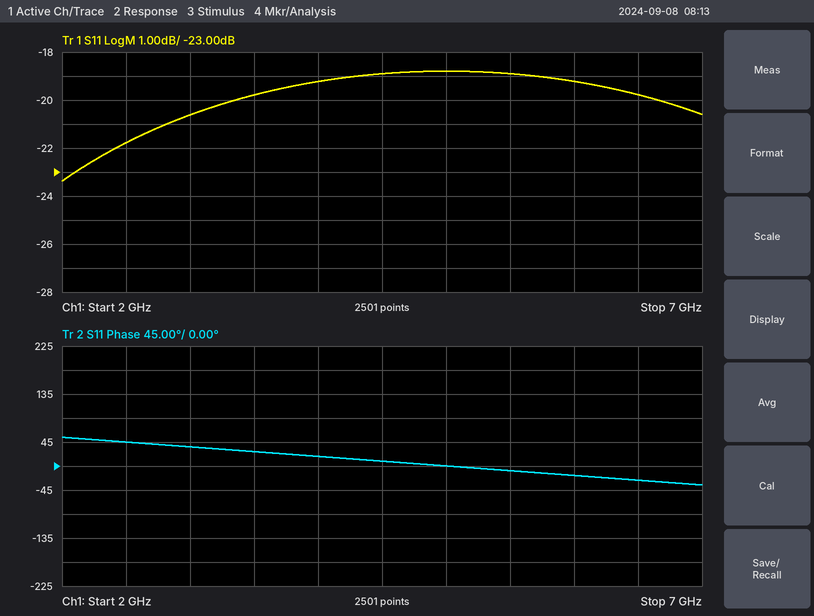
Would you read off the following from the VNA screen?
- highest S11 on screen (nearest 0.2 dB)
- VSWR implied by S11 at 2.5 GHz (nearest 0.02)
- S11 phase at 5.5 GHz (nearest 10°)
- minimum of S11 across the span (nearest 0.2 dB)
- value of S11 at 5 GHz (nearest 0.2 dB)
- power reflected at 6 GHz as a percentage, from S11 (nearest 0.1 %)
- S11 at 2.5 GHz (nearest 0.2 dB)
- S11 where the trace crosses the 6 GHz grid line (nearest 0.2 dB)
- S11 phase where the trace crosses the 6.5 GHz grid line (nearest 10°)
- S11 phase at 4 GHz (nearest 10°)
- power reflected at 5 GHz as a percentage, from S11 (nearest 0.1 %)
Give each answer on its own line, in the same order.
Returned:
-18.8 dB
1.18
-10°
-23.4 dB
-18.8 dB
1.2 %
-21.8 dB
-19.2 dB
-30°
20°
1.3 %
